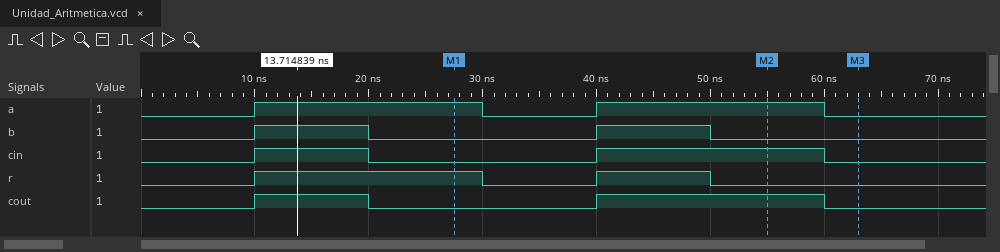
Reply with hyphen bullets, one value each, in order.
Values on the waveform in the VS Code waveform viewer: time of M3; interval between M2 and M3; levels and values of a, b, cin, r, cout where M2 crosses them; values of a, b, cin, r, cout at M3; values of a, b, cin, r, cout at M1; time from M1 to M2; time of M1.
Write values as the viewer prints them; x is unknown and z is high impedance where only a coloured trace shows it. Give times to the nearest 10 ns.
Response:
- 60 ns
- 10 ns
- a=1, b=0, cin=1, r=0, cout=1
- a=0, b=0, cin=0, r=0, cout=0
- a=1, b=0, cin=0, r=1, cout=0
- 30 ns
- 30 ns
